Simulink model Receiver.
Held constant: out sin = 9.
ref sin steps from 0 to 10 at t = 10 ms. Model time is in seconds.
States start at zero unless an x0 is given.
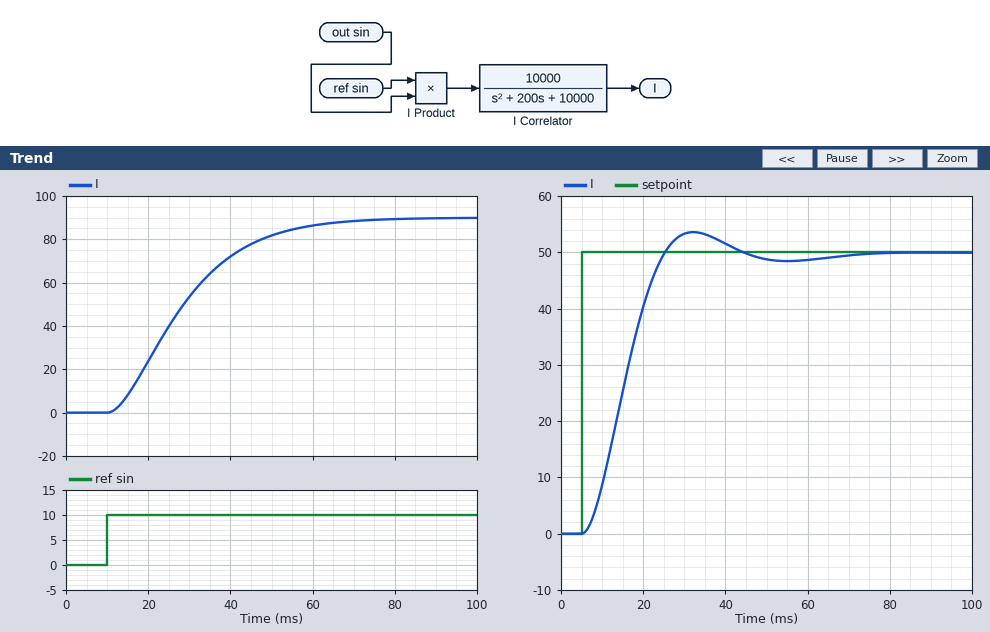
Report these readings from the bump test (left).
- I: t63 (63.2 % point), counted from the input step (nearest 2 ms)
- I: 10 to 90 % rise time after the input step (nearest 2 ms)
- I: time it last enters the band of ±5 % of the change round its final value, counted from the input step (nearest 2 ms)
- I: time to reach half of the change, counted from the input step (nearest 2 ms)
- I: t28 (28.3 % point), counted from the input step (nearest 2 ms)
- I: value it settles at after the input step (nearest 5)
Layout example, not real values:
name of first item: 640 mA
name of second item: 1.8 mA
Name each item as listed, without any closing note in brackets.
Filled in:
I: t63 (63.2 % point), counted from the input step: 22 ms
I: 10 to 90 % rise time after the input step: 34 ms
I: time it last enters the band of ±5 % of the change round its final value, counted from the input step: 48 ms
I: time to reach half of the change, counted from the input step: 16 ms
I: t28 (28.3 % point), counted from the input step: 10 ms
I: value it settles at after the input step: 90
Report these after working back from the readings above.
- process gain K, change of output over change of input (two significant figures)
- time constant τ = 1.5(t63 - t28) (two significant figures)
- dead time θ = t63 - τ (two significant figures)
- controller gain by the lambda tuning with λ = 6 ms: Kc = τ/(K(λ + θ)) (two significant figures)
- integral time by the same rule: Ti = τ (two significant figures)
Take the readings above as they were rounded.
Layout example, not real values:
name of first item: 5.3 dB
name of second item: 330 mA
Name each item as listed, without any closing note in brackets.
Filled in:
process gain K, change of output over change of input: 9.0
time constant τ = 1.5(t63 - t28): 18 ms
dead time θ = t63 - τ: 4.0 ms
controller gain by the lambda tuning with λ = 6 ms: Kc = τ/(K(λ + θ)): 0.20
integral time by the same rule: Ti = τ: 18 ms
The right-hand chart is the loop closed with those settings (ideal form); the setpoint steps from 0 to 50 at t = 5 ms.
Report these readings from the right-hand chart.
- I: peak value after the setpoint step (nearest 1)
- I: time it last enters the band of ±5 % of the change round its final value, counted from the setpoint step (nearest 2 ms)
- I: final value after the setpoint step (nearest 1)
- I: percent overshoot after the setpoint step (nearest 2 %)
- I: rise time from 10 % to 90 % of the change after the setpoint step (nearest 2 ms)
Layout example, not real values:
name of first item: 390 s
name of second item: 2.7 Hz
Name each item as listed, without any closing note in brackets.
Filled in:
I: peak value after the setpoint step: 54
I: time it last enters the band of ±5 % of the change round its final value, counted from the setpoint step: 32 ms
I: final value after the setpoint step: 50
I: percent overshoot after the setpoint step: 8 %
I: rise time from 10 % to 90 % of the change after the setpoint step: 14 ms
